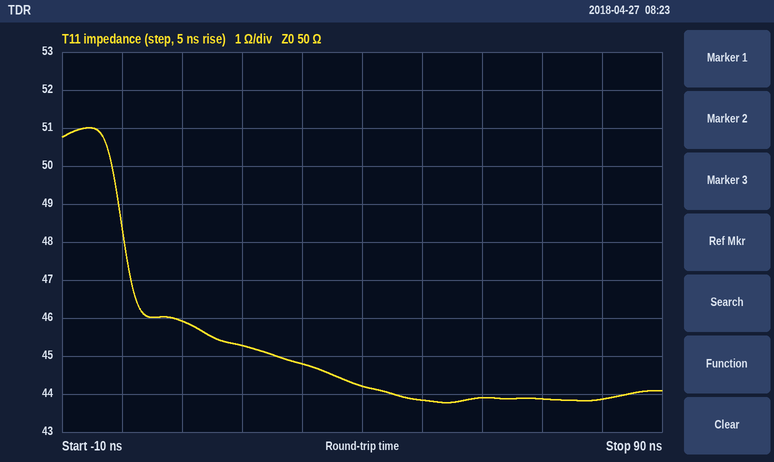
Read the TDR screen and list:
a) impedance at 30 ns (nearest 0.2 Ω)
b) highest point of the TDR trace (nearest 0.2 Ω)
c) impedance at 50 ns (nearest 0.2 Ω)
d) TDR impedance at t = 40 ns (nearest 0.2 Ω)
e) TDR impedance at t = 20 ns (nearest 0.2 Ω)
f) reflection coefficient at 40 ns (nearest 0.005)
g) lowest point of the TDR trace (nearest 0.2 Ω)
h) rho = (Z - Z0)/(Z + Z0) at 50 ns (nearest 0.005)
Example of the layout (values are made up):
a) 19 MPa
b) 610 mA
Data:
a) 44.8 Ω
b) 51.0 Ω
c) 43.8 Ω
d) 44.2 Ω
e) 45.2 Ω
f) -0.060
g) 43.8 Ω
h) -0.065
